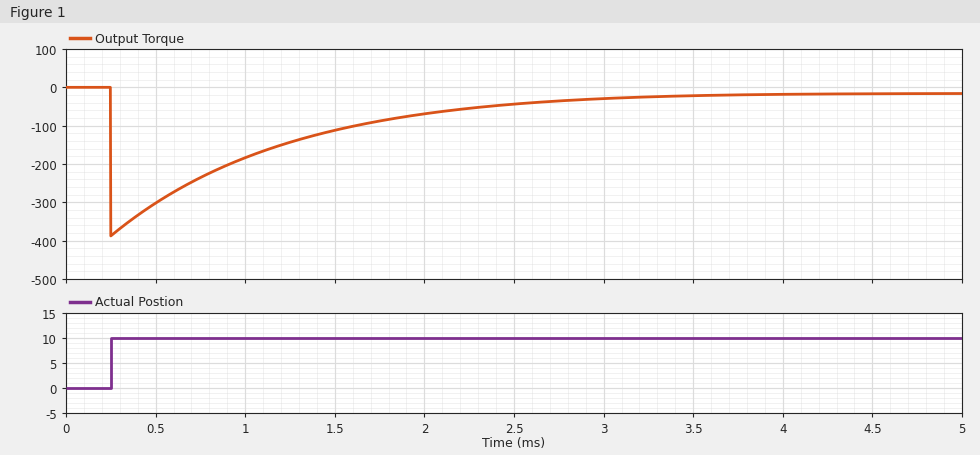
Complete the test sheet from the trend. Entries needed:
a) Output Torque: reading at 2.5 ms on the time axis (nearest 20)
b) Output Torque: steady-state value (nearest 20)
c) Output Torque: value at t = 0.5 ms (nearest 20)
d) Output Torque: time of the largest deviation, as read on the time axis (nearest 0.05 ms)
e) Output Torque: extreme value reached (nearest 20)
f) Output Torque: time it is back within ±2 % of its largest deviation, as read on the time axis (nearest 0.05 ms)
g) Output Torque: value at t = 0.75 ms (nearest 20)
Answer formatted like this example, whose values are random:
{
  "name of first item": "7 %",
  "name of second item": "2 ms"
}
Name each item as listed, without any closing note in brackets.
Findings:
{
  "Output Torque: reading at 2.5 ms on the time axis": "-40",
  "Output Torque: steady-state value": "-20",
  "Output Torque: value at t = 0.5 ms": "-300",
  "Output Torque: time of the largest deviation, as read on the time axis": "0.25 ms",
  "Output Torque: extreme value reached": "-380",
  "Output Torque: time it is back within ±2 % of its largest deviation, as read on the time axis": "3.35 ms",
  "Output Torque: value at t = 0.75 ms": "-240"
}
